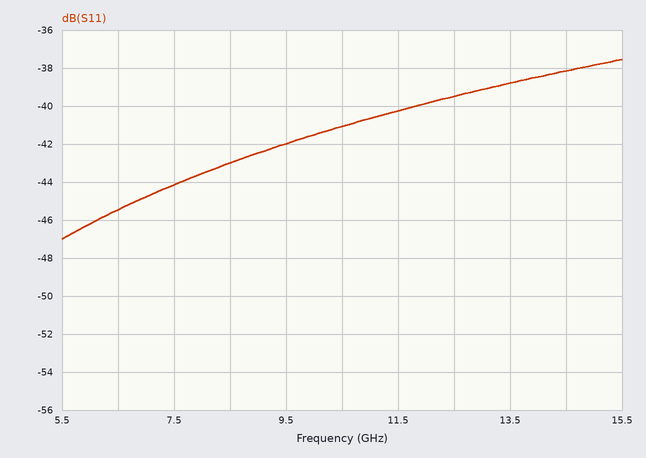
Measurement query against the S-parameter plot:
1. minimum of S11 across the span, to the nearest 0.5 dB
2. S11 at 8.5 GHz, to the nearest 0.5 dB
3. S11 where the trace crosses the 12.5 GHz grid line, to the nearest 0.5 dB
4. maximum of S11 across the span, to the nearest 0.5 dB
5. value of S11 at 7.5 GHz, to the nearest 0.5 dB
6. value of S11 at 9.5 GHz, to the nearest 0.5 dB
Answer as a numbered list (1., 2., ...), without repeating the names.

1. -47.0 dB
2. -43.0 dB
3. -39.5 dB
4. -37.5 dB
5. -44.0 dB
6. -42.0 dB
